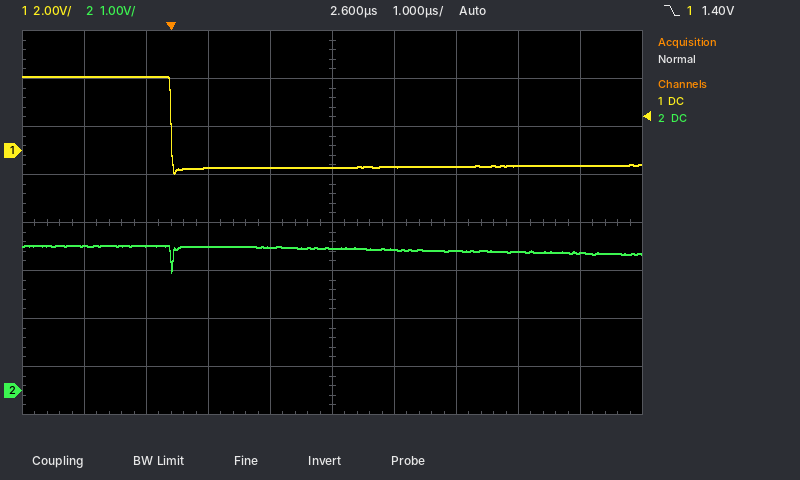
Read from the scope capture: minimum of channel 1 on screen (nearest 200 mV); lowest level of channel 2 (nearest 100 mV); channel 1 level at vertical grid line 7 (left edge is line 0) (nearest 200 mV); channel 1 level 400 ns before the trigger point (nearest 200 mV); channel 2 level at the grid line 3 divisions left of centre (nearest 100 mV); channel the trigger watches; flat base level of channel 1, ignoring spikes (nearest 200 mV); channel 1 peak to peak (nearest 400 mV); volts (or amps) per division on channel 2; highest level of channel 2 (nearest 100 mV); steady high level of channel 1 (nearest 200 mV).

-1.0 V
2.5 V
-600 mV
3.0 V
3.0 V
channel 1
-600 mV
4.0 V
1 V
3.0 V
3.0 V
